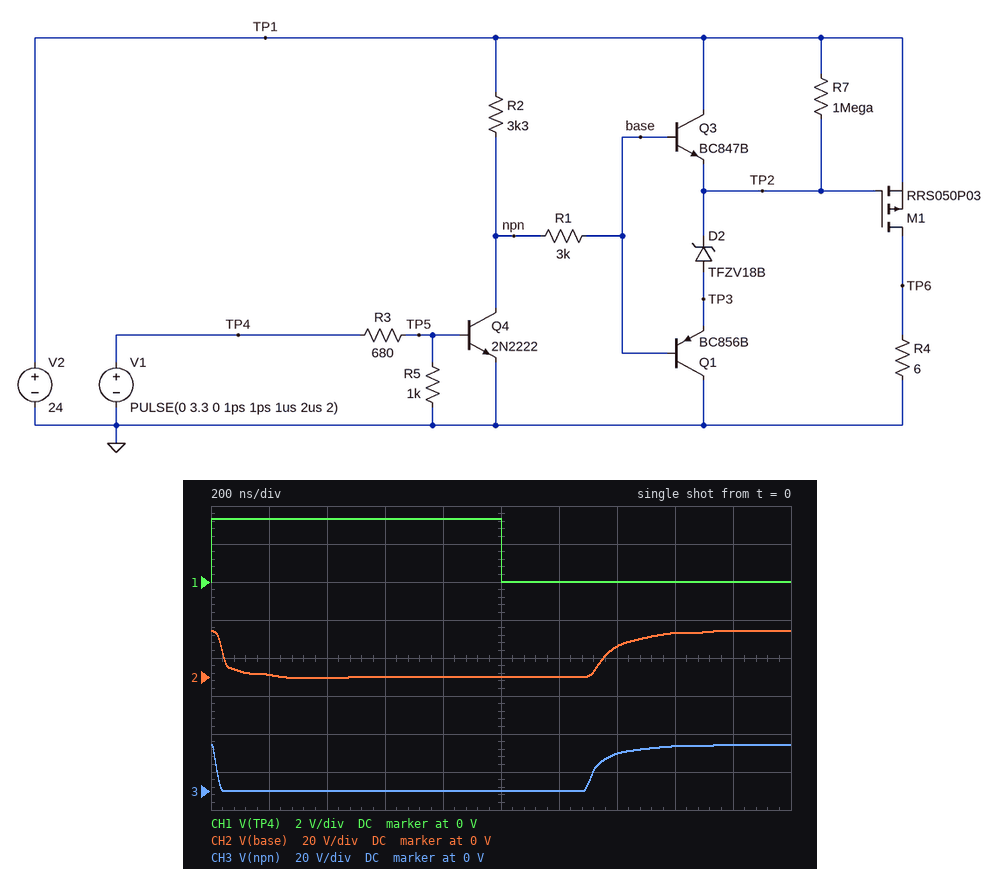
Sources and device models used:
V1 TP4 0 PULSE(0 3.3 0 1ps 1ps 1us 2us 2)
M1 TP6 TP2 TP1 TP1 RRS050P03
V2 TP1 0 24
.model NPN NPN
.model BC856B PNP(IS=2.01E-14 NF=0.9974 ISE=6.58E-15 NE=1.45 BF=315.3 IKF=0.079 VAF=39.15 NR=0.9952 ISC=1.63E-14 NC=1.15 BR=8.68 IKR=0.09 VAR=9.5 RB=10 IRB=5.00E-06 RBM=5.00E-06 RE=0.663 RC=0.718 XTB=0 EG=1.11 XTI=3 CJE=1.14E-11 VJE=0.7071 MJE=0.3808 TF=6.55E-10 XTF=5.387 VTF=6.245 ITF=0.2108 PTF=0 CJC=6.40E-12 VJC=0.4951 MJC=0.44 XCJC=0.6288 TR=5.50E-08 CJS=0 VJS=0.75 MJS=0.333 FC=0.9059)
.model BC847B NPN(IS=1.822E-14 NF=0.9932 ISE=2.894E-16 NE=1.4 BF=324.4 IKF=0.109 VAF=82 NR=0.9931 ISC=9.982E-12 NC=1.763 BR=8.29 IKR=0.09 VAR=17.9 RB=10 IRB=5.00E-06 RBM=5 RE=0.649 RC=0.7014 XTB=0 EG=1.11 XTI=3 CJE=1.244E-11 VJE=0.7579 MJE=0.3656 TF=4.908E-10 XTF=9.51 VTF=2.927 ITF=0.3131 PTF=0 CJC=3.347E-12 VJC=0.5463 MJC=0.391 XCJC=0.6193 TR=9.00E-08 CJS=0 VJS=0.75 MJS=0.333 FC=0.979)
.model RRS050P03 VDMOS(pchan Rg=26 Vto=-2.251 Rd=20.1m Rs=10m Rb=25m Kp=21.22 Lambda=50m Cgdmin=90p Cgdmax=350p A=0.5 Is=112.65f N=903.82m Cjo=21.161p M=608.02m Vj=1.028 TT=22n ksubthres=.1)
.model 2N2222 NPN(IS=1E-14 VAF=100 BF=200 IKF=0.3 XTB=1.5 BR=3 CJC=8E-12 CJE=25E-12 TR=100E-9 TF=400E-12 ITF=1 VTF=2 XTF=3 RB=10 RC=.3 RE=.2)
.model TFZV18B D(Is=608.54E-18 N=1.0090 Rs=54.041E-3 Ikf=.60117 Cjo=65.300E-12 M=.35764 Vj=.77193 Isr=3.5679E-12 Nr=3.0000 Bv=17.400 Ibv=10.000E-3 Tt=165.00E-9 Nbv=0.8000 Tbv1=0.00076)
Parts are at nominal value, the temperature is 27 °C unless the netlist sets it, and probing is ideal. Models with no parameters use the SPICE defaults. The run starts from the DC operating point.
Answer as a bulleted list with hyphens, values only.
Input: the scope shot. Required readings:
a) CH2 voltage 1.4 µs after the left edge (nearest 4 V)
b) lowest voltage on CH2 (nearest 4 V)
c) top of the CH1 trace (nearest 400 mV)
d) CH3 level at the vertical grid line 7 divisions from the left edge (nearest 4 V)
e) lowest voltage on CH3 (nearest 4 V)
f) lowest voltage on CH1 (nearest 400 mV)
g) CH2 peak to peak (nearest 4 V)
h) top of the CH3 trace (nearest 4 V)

- 16 V
- 0 V
- 3.2 V
- 20 V
- 0 V
- 0 V
- 24 V
- 24 V
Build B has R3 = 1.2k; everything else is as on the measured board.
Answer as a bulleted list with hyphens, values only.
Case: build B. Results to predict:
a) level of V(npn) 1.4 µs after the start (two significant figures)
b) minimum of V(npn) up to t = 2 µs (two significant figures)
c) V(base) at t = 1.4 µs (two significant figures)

- 22 V
- 28 mV
- 20 V
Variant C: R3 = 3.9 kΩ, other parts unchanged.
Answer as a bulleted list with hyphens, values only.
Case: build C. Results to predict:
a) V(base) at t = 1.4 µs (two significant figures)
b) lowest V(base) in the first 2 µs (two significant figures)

- 24 V
- 19 V
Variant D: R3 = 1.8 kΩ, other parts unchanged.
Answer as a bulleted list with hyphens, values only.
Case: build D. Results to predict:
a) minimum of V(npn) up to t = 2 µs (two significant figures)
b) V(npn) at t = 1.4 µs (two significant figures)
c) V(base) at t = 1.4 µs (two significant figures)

- 42 mV
- 23 V
- 22 V
